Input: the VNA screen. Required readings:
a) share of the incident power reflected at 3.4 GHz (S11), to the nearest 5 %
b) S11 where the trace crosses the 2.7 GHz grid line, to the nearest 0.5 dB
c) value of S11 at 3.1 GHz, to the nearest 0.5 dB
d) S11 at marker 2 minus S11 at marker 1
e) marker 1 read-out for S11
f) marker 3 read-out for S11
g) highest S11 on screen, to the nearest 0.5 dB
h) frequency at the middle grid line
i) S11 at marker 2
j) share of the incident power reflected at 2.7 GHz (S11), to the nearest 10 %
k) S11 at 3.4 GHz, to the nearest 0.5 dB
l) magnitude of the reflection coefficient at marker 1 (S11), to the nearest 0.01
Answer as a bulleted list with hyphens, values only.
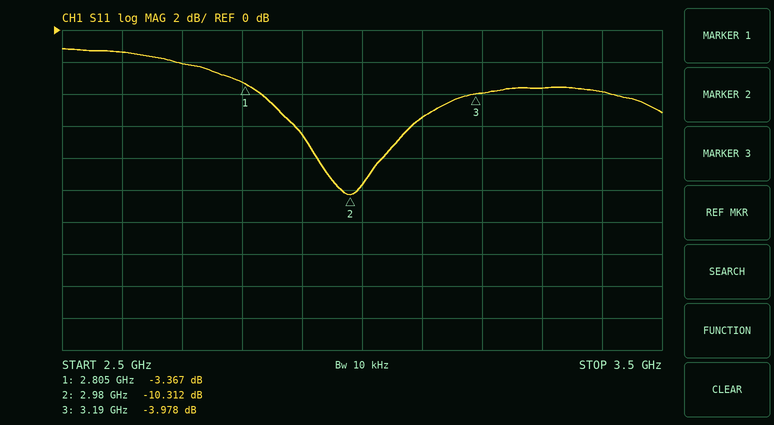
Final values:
- 40 %
- -2.0 dB
- -5.5 dB
- -6.945 dB
- -3.367 dB
- -3.978 dB
- -1.0 dB
- 3 GHz
- -10.312 dB
- 60 %
- -4.0 dB
- 0.68
